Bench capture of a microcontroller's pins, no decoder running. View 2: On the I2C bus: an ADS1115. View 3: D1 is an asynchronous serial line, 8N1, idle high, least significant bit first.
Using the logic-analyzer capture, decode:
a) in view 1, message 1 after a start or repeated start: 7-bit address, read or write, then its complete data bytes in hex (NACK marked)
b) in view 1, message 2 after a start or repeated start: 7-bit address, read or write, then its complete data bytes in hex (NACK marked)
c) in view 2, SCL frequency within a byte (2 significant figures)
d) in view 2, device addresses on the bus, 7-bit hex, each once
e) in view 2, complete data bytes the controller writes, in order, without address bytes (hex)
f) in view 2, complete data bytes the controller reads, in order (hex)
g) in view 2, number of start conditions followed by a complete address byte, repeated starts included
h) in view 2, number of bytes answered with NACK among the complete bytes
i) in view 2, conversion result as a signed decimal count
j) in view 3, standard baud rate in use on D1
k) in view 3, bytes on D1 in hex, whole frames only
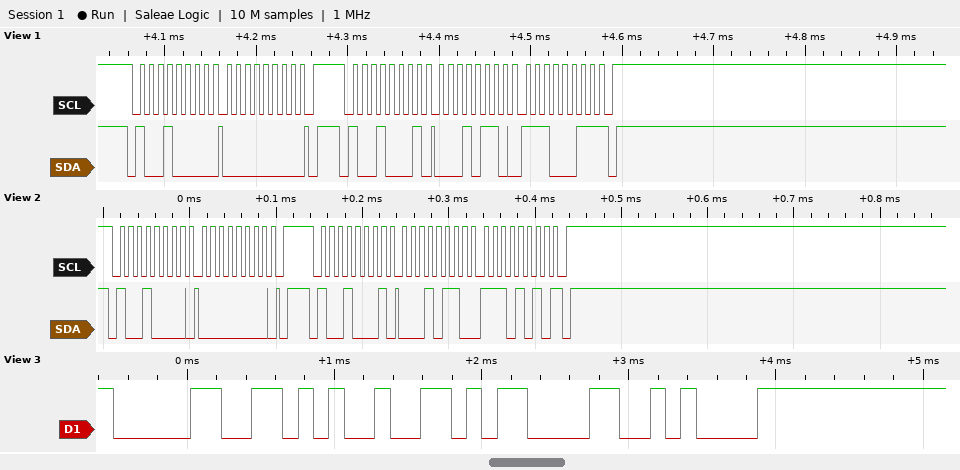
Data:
0x48 write: 00
0x48 read: 16 E3 NACK
100 kHz
0x48
00
16 EA
2
1
5866
9600 baud
0x30 0x25 0x0D 0x0A
